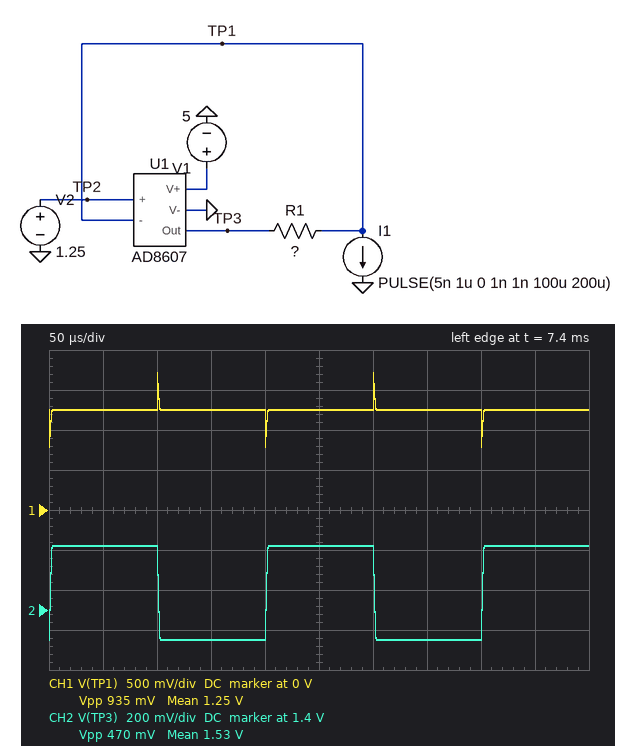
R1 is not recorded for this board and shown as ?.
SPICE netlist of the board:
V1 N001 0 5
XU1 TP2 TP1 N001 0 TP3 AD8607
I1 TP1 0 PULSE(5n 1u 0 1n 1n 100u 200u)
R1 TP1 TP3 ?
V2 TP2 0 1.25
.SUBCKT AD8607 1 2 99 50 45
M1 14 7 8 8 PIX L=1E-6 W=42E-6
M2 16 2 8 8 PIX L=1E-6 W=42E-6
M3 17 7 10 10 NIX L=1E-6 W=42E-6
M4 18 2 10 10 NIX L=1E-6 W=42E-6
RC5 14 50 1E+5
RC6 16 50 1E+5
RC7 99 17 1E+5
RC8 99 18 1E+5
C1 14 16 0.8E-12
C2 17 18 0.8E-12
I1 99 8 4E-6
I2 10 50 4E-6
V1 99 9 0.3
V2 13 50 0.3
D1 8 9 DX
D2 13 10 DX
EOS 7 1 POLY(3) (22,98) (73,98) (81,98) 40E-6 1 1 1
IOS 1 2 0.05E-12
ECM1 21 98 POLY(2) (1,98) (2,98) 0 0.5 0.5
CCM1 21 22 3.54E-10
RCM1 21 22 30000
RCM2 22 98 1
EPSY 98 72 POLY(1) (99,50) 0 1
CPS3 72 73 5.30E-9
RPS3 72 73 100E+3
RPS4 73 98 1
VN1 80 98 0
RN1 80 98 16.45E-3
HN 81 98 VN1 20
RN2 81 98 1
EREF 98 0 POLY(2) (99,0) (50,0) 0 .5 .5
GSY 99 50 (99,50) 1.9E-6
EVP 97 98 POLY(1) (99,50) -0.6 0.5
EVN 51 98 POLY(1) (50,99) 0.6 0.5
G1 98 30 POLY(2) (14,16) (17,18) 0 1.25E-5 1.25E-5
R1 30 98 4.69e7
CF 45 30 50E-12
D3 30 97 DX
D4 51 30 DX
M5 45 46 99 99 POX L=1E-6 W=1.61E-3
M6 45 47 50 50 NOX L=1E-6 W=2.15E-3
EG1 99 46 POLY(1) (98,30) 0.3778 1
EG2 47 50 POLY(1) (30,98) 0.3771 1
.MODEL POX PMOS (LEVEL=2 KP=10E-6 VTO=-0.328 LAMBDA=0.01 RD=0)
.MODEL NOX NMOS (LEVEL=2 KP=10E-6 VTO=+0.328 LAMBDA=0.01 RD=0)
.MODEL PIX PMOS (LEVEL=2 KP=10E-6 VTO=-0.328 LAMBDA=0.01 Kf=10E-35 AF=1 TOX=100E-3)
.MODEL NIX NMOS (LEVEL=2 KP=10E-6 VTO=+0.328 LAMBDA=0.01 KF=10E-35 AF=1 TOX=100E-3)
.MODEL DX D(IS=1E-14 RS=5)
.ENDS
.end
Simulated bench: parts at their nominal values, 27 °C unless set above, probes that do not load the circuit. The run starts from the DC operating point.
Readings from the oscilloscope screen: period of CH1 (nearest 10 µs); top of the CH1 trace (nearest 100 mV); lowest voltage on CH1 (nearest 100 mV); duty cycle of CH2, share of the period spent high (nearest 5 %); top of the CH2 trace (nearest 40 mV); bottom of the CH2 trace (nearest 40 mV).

200 µs
1.7 V
800 mV
50 %
1.72 V
1.24 V
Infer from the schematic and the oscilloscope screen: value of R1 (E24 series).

470 kΩ
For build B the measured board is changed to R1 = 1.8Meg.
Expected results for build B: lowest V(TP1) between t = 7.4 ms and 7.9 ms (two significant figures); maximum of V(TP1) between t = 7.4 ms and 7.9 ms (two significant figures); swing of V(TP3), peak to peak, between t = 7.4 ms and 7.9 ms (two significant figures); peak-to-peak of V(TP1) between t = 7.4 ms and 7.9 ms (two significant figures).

-540 mV
3.0 V
1.8 V
3.6 V
